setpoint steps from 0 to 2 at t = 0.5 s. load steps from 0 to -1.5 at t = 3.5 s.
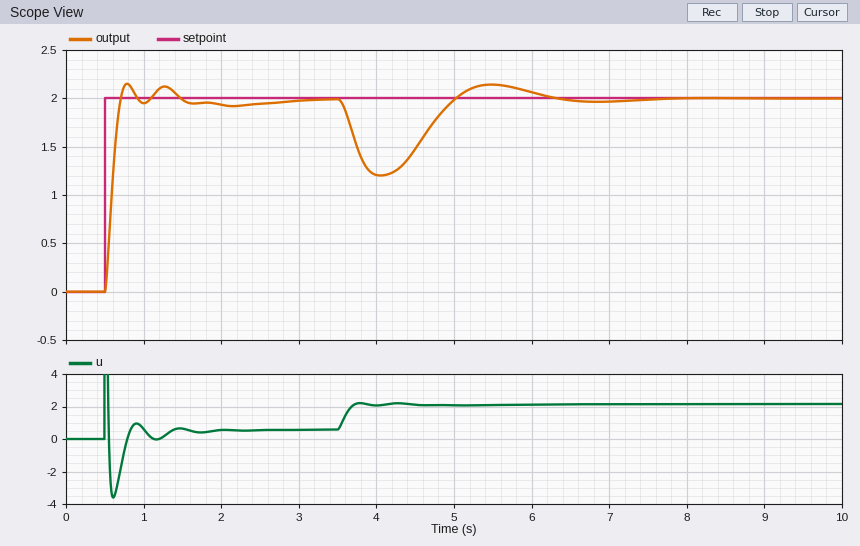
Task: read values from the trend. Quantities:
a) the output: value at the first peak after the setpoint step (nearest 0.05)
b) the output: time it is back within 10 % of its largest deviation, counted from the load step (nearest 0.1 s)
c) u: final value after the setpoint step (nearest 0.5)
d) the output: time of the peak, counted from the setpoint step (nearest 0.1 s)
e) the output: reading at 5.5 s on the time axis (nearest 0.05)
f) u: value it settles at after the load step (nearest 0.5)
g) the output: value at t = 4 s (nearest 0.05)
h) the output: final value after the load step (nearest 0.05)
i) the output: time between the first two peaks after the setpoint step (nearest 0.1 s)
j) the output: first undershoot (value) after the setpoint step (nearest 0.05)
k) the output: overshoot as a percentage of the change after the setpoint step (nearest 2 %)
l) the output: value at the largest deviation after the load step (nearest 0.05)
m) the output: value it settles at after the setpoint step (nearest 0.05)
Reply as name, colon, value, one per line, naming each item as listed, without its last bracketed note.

the output: value at the first peak after the setpoint step: 2.15
the output: time it is back within 10 % of its largest deviation, counted from the load step: 2.4 s
u: final value after the setpoint step: 0.5
the output: time of the peak, counted from the setpoint step: 0.3 s
the output: reading at 5.5 s on the time axis: 2.15
u: value it settles at after the load step: 2.0
the output: value at t = 4 s: 1.20
the output: final value after the load step: 2.00
the output: time between the first two peaks after the setpoint step: 0.5 s
the output: first undershoot (value) after the setpoint step: 1.95
the output: overshoot as a percentage of the change after the setpoint step: 8 %
the output: value at the largest deviation after the load step: 1.20
the output: value it settles at after the setpoint step: 2.00
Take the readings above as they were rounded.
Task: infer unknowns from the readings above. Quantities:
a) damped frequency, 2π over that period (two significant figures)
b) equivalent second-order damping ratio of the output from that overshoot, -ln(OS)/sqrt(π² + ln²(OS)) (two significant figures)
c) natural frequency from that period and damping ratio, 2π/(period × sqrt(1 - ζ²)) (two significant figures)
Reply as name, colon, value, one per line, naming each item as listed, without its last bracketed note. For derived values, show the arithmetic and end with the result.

damped frequency, 2π over that period: 2π / 0.5 = 13 rad/s
equivalent second-order damping ratio of the output from that overshoot, -ln(OS)/sqrt(π² + ln²(OS)): ln(0.08) = -2.526; 2.526 / sqrt(9.870 + 6.379) = 0.63
natural frequency from that period and damping ratio, 2π/(period × sqrt(1 - ζ²)): 2π / (0.5 × sqrt(1 - 0.63²)) = 16 rad/s
